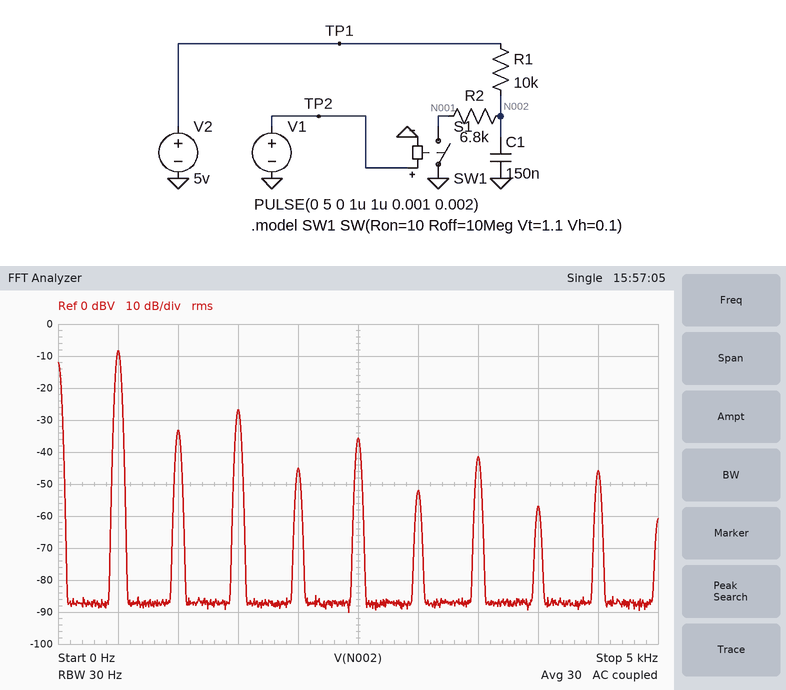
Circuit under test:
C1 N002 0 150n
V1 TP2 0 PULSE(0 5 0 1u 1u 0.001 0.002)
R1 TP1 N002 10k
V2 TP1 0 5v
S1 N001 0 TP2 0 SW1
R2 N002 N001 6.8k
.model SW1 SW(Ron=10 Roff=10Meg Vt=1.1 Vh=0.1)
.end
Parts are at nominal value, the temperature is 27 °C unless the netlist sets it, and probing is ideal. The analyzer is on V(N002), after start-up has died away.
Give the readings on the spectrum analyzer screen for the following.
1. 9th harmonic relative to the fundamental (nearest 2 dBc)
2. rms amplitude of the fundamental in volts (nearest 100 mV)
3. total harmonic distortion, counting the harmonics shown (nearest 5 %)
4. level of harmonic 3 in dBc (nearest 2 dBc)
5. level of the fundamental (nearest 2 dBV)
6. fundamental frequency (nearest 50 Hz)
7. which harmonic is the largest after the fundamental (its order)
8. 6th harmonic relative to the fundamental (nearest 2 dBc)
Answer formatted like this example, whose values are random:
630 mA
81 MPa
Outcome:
-38 dBc
400 mV
15 %
-18 dBc
-8 dBV
500 Hz
3
-44 dBc
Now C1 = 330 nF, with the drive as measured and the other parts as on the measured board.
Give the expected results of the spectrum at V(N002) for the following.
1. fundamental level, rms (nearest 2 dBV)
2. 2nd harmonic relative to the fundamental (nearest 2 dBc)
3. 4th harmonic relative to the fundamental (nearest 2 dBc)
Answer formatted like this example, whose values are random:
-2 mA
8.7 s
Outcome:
-14 dBV
-32 dBc
-44 dBc
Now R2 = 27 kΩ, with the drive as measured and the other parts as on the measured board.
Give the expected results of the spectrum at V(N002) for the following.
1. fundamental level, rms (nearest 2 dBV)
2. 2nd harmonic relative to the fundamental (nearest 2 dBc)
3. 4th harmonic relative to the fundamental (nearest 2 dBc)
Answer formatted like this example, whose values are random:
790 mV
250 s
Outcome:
-16 dBV
-36 dBc
-48 dBc
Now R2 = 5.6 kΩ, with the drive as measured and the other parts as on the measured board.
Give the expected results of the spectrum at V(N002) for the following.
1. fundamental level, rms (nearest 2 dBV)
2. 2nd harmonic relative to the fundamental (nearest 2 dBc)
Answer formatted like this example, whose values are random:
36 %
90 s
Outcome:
-8 dBV
-24 dBc
